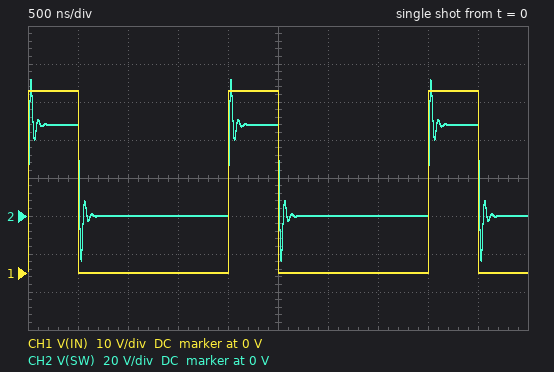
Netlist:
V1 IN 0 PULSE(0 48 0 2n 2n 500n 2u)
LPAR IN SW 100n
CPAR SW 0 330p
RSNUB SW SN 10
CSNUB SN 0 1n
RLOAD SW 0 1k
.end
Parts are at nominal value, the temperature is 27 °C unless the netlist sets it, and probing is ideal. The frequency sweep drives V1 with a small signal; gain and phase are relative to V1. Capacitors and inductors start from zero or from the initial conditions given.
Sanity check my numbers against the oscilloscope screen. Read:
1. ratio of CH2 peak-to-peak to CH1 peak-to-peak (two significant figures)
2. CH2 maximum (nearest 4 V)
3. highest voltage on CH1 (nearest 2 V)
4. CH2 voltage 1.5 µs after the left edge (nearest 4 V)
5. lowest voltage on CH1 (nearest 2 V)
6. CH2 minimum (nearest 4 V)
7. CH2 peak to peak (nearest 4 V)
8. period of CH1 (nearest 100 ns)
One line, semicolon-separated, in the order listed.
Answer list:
2.0; 72 V; 48 V; 0 V; 0 V; -24 V; 96 V; 2.0 µs
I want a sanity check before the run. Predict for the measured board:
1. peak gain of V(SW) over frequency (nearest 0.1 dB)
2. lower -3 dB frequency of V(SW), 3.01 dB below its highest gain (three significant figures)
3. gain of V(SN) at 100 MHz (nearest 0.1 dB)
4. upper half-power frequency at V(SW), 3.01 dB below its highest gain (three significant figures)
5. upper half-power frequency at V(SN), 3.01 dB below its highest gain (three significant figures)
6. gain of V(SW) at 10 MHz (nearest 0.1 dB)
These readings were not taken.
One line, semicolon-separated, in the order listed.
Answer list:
6.0 dB; 8.31 MHz; -39.2 dB; 18.9 MHz; 17.6 MHz; 4.2 dB
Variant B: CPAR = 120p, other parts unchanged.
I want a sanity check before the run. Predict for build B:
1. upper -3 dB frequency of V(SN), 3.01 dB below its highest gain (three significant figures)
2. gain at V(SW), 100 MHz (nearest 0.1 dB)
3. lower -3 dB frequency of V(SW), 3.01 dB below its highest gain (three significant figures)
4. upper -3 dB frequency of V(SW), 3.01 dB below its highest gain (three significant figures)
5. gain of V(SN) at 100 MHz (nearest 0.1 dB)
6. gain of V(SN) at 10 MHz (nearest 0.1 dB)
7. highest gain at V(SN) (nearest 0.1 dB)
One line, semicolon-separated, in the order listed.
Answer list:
18.6 MHz; -17.8 dB; 5.83 MHz; 21.0 MHz; -33.9 dB; 1.7 dB; 2.0 dB
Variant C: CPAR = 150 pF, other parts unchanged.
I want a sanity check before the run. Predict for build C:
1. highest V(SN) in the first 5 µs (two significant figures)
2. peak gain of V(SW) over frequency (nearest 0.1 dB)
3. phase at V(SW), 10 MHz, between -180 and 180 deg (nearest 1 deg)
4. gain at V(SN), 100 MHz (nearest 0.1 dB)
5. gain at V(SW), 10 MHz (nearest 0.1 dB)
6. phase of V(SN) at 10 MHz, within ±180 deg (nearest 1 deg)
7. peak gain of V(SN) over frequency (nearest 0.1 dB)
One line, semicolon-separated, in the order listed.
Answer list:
59 V; 4.5 dB; -16 deg; -34.7 dB; 3.3 dB; -48 deg; 2.2 dB
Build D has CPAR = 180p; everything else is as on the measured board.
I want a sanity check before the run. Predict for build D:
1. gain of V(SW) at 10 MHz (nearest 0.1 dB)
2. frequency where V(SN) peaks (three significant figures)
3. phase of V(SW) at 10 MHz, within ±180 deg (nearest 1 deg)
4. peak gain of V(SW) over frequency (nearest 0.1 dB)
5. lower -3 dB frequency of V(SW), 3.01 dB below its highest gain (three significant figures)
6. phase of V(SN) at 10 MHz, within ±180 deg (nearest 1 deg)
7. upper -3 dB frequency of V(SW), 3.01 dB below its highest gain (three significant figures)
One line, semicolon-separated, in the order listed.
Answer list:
3.5 dB; 12.6 MHz; -16 deg; 4.8 dB; 6.76 MHz; -48 deg; 20.5 MHz
